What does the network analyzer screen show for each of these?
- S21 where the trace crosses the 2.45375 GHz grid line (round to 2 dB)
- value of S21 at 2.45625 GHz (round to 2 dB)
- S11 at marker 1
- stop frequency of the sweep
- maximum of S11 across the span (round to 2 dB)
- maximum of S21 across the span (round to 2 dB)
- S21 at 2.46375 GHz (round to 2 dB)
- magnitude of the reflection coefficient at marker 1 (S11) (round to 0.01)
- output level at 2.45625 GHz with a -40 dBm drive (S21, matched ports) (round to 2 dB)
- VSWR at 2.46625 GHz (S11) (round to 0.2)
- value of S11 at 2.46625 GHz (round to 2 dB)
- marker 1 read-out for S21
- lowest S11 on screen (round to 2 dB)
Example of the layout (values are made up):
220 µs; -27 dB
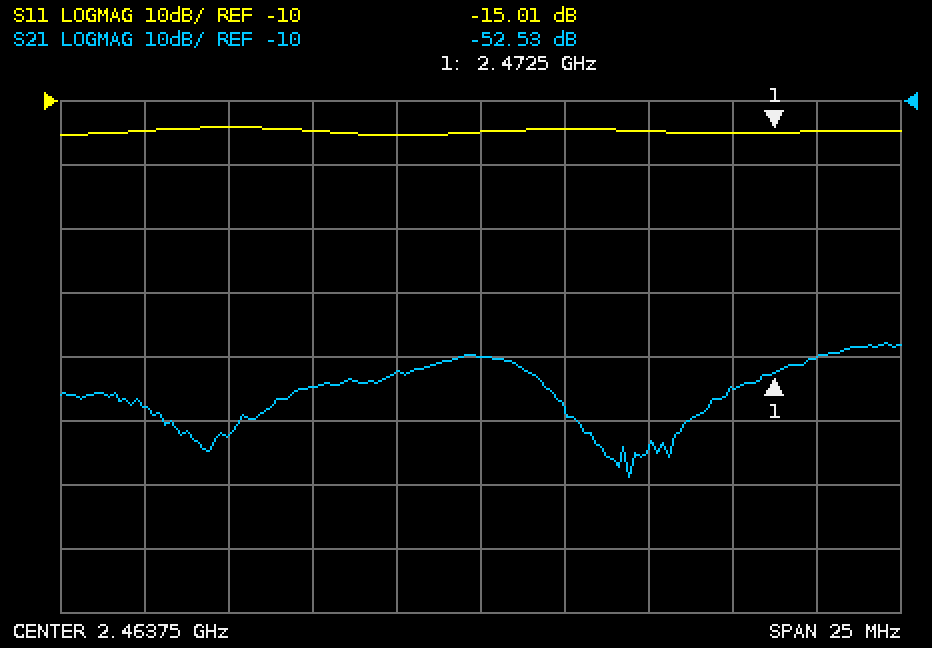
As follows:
-58 dB; -62 dB; -15.01 dB; 2.47625 GHz; -14 dB; -48 dB; -50 dB; 0.18; -102 dBm; 1.4; -14 dB; -52.53 dB; -16 dB
